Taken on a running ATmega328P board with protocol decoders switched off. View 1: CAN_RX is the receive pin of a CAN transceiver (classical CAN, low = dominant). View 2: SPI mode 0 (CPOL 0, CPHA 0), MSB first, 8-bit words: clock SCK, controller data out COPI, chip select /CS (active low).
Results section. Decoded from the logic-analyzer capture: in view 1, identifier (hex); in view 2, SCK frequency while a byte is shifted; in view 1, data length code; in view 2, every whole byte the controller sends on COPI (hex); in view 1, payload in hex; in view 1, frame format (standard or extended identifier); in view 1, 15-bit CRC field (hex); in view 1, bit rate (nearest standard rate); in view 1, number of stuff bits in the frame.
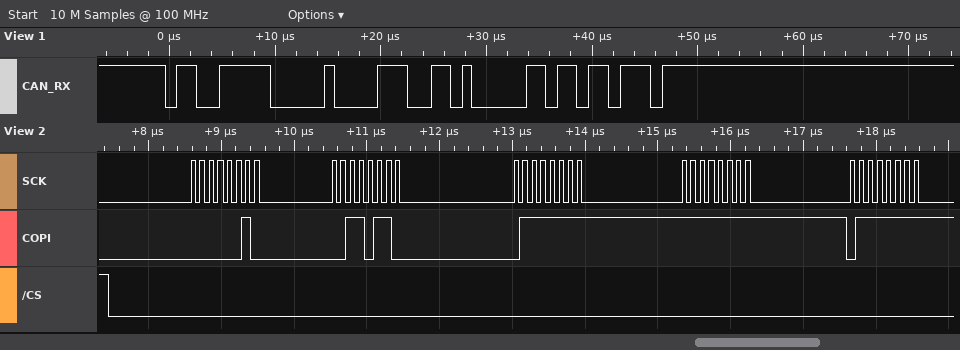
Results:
0x67C
8 MHz
1
02 36 7F FF 7F
CD
standard
0x02DB
1000 kbit/s
3
